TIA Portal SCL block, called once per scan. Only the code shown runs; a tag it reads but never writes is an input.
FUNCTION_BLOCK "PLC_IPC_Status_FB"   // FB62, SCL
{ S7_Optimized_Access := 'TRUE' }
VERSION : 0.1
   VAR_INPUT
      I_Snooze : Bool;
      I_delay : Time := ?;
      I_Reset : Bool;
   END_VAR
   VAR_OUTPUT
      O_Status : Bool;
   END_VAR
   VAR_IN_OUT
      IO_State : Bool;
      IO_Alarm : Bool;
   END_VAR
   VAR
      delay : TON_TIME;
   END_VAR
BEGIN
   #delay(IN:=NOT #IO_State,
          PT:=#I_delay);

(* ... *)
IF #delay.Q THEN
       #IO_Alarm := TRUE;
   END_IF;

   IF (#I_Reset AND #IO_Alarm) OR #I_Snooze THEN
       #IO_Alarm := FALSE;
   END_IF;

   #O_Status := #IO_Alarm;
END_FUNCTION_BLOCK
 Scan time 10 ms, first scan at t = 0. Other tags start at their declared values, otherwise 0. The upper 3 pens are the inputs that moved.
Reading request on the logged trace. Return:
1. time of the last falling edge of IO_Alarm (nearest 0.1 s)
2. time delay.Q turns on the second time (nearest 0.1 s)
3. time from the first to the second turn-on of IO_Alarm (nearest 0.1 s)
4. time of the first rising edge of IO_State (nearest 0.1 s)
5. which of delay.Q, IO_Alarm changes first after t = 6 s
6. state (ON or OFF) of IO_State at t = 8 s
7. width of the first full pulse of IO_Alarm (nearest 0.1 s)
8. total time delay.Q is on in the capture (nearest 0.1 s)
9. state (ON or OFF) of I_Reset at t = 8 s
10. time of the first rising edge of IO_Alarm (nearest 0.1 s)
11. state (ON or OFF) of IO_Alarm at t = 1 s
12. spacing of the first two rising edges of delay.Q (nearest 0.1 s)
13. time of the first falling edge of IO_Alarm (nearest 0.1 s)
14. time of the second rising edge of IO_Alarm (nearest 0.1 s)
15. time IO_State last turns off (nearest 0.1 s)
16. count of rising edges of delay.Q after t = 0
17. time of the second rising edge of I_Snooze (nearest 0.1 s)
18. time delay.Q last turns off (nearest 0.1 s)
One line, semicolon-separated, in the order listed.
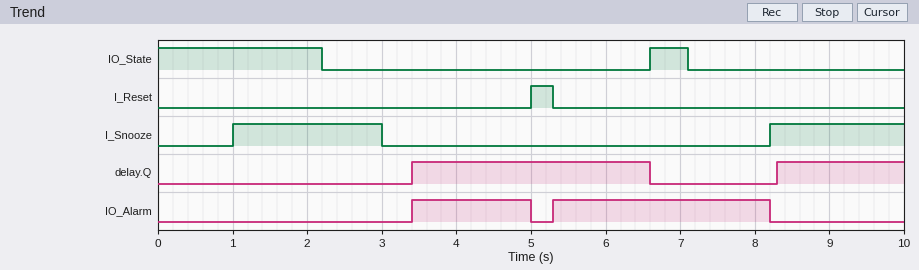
8.2 s; 8.3 s; 1.9 s; 6.6 s; delay.Q; OFF; 1.6 s; 4.9 s; OFF; 3.4 s; OFF; 4.9 s; 5.0 s; 5.3 s; 7.1 s; 2; 8.2 s; 6.6 s
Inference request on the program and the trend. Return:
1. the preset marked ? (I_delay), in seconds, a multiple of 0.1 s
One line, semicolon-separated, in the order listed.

1.2 s
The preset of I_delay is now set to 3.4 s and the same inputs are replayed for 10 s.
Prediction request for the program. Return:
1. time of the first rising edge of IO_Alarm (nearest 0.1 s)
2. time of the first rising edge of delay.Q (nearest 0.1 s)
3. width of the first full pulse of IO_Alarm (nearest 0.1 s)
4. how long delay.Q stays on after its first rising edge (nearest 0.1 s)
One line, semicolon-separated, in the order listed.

5.6 s; 5.6 s; 2.6 s; 1.0 s
